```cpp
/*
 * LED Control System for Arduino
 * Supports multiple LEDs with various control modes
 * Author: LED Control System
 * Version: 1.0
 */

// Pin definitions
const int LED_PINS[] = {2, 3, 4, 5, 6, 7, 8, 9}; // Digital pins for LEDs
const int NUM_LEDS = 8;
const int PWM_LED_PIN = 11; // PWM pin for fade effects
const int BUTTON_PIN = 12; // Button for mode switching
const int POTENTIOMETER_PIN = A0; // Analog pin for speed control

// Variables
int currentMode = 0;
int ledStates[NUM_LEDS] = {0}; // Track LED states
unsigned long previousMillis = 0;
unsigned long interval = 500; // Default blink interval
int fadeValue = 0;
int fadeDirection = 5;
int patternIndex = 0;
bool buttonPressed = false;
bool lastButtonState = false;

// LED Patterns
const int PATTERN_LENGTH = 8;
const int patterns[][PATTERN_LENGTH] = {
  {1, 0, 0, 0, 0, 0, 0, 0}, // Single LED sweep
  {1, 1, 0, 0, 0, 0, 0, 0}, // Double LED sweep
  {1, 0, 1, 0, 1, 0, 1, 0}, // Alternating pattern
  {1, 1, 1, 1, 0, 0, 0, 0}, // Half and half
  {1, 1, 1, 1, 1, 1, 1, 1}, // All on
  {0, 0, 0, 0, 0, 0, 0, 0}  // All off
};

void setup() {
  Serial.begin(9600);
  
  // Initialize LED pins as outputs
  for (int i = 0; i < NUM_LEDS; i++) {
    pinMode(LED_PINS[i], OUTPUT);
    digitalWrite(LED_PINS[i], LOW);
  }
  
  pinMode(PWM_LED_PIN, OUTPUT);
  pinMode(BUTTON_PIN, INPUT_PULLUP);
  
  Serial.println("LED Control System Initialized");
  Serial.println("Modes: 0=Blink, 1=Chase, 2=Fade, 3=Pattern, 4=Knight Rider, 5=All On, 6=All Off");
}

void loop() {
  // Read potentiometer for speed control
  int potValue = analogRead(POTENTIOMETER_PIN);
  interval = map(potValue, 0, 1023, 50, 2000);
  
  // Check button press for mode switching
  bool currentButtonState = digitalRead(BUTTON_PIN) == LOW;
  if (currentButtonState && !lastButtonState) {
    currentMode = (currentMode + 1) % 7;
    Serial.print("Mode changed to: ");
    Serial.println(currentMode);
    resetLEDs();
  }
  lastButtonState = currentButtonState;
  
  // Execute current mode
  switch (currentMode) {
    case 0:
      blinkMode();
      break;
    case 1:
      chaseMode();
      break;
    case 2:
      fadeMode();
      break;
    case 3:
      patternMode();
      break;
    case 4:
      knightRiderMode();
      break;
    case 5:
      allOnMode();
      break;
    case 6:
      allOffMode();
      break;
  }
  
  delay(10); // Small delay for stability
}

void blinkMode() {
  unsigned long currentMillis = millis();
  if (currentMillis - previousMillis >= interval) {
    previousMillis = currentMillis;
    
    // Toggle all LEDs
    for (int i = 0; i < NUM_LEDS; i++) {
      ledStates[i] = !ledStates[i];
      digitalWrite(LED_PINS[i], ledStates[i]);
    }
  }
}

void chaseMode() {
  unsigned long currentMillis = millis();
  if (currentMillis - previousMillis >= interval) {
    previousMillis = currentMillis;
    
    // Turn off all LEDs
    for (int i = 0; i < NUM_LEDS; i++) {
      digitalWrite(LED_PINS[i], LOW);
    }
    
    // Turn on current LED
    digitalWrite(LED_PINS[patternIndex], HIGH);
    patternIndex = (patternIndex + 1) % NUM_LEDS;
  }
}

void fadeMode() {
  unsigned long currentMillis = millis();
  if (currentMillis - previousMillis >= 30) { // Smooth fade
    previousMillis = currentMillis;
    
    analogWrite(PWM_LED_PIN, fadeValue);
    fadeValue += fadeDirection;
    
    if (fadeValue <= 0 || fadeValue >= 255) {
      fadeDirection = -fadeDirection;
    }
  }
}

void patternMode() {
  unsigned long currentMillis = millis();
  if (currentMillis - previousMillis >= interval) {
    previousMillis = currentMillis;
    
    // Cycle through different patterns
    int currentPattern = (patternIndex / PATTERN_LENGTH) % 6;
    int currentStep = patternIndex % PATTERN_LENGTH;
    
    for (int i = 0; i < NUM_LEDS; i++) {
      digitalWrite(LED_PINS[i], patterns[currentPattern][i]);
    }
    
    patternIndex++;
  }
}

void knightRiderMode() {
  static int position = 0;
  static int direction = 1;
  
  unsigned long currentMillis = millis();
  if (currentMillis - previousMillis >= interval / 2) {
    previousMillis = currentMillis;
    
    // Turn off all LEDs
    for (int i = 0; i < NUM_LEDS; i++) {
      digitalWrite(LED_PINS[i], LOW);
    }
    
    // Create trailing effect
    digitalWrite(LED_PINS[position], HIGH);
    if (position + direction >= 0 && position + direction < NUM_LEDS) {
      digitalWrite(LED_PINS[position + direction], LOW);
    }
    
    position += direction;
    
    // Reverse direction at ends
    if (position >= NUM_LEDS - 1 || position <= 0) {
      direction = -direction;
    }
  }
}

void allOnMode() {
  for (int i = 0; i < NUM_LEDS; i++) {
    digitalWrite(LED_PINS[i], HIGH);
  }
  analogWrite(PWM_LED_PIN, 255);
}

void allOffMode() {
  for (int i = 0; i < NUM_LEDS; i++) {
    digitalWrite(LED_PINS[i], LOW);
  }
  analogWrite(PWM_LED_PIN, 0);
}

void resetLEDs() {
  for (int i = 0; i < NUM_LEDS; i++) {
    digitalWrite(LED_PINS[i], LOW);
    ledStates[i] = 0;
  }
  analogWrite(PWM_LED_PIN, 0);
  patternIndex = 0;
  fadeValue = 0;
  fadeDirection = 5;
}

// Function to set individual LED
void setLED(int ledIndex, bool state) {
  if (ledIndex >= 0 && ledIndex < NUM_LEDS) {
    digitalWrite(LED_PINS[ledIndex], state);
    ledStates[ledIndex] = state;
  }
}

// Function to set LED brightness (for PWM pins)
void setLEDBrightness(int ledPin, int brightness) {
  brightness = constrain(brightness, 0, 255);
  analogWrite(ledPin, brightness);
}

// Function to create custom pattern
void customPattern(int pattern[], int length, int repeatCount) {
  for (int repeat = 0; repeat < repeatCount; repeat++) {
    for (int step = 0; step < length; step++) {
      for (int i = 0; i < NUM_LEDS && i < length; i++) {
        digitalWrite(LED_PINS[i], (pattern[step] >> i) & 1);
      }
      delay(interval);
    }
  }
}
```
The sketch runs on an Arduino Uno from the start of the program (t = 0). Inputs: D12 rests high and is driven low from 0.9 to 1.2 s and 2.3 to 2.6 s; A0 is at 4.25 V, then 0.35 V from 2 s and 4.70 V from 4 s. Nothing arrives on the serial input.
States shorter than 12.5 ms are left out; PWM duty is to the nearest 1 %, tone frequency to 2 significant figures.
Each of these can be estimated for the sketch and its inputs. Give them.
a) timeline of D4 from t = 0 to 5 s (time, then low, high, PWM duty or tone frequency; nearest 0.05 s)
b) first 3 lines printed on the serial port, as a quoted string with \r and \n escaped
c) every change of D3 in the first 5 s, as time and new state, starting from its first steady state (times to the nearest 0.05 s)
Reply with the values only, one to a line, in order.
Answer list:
0 s low; 2.2 s high; 2.3 s low
"LED Control System Initialized\r\nModes: 0=Blink, 1=Chase, 2=Fade, 3=Pattern, 4=Knight Rider, 5=All On, 6=All Off\r\nMode changed to: 1\r\n"
0 s low; 2 s high; 2.2 s low
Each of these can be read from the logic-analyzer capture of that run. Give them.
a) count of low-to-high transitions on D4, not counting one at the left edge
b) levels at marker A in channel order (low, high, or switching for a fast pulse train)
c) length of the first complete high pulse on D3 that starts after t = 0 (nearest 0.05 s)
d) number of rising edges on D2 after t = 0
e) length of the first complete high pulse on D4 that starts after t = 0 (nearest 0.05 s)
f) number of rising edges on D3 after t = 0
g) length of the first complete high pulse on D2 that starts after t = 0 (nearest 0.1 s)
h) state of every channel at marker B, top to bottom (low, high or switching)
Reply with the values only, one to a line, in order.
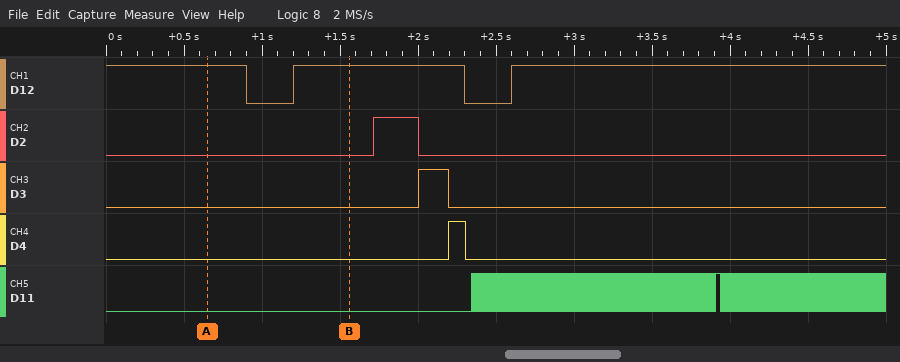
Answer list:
1
D12 high, D2 low, D3 low, D4 low, D11 low
0.20 s
1
0.10 s
1
0.3 s
D12 high, D2 low, D3 low, D4 low, D11 low
